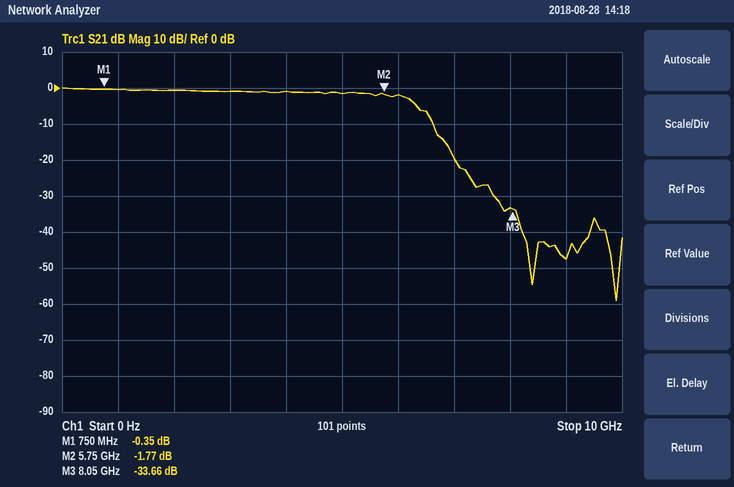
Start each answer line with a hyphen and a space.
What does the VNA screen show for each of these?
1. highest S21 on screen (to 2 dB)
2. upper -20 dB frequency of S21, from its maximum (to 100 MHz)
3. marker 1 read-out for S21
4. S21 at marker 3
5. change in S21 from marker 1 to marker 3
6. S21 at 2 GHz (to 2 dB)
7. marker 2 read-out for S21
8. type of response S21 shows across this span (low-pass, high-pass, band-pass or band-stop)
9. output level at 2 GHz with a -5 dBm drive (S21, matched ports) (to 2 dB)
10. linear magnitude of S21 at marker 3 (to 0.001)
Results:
- 0 dB
- 7.0 GHz
- -0.35 dB
- -33.66 dB
- -33.31 dB
- 0 dB
- -1.77 dB
- low-pass
- -6 dBm
- 0.021
